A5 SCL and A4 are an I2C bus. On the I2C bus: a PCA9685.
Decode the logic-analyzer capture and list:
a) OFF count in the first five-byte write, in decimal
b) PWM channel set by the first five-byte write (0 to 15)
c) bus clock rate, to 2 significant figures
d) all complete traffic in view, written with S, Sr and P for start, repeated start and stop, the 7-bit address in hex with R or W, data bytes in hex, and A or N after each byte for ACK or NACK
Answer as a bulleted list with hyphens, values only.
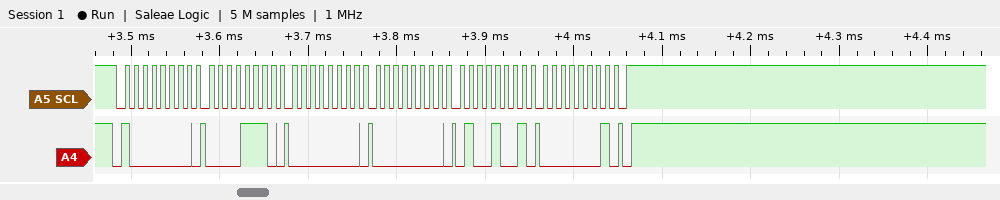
- 329
- 2
- 100 kHz
- S 40W A 0E A 00 A 00 A 49 A 01 A P
